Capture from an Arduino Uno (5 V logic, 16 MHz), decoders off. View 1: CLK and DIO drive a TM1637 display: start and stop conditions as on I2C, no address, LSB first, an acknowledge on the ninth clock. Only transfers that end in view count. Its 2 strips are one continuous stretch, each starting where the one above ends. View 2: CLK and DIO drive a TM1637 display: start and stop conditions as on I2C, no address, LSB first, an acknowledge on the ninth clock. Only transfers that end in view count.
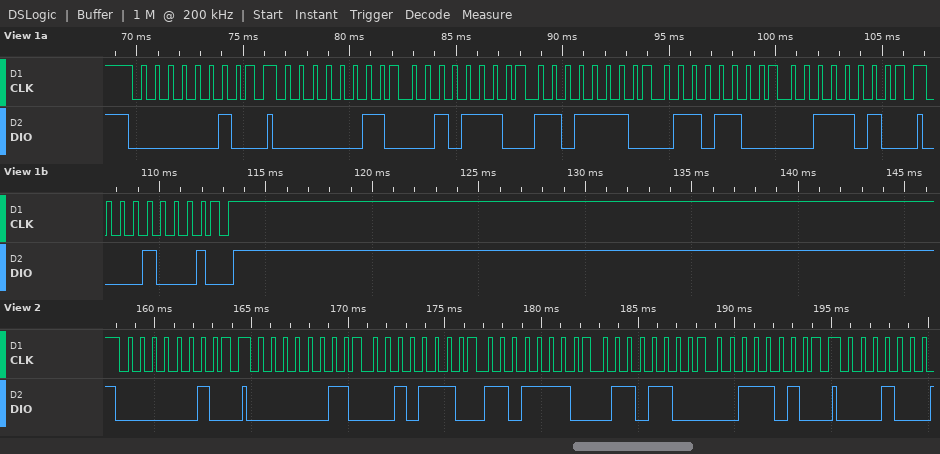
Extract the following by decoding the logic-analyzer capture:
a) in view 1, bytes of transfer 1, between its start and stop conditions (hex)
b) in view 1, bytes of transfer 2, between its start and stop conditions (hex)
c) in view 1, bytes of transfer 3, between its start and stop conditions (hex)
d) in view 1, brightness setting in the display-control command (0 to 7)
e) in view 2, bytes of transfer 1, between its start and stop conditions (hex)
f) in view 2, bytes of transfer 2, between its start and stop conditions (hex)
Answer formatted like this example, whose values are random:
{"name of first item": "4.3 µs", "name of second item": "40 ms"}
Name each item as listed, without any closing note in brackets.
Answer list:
{"in view 1, bytes of transfer 1, between its start and stop conditions": "40", "in view 1, bytes of transfer 2, between its start and stop conditions": "C0 74 7B 36 5C", "in view 1, bytes of transfer 3, between its start and stop conditions": "88", "in view 1, brightness setting in the display-control command": "0", "in view 2, bytes of transfer 1, between its start and stop conditions": "40", "in view 2, bytes of transfer 2, between its start and stop conditions": "C0 74 7B 36 5C"}
